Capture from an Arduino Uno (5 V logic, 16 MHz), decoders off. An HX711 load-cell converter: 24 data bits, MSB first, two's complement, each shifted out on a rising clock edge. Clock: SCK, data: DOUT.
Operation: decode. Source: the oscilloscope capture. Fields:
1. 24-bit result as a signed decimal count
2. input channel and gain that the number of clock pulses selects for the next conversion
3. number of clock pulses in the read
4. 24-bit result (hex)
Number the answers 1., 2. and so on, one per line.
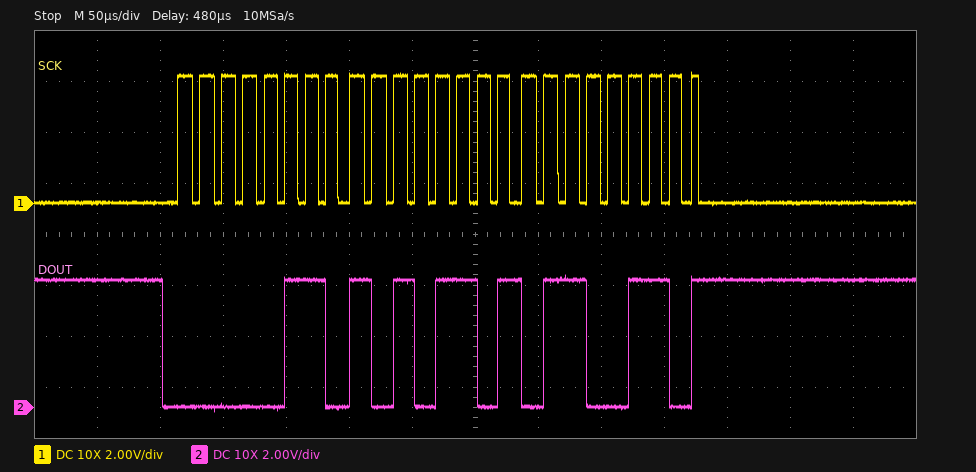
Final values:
1. 437606
2. channel A, gain 128
3. 25
4. 0x06AD66
